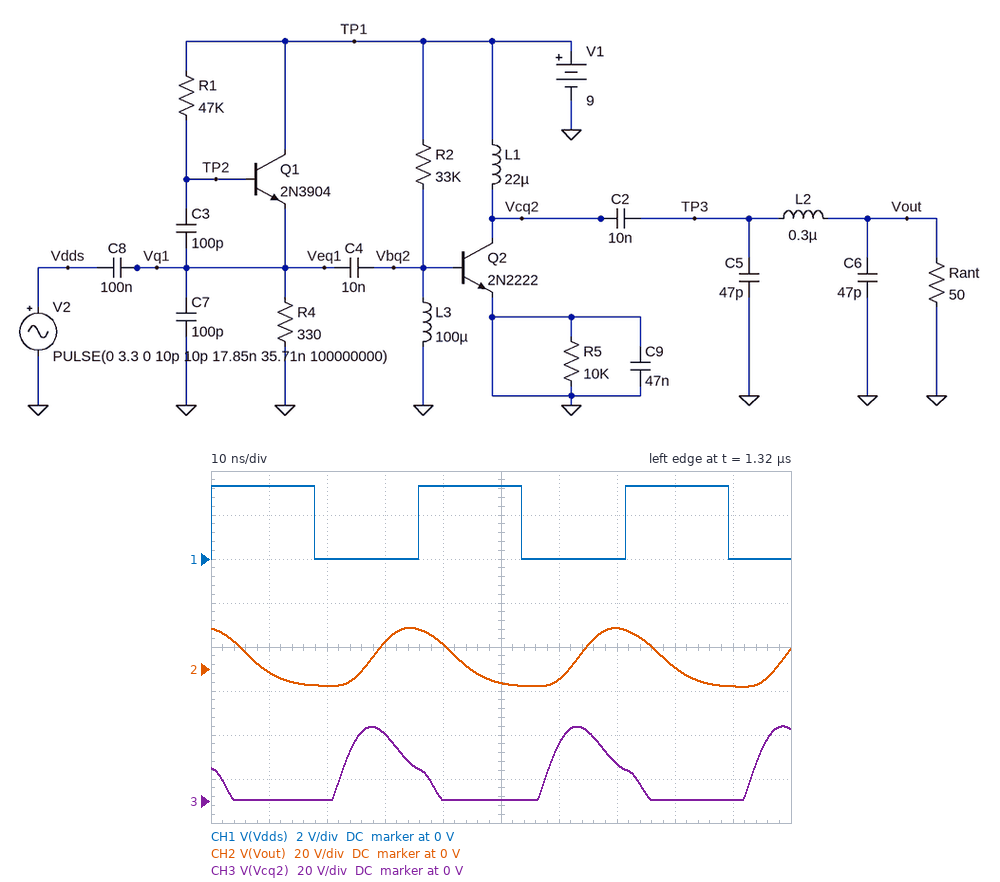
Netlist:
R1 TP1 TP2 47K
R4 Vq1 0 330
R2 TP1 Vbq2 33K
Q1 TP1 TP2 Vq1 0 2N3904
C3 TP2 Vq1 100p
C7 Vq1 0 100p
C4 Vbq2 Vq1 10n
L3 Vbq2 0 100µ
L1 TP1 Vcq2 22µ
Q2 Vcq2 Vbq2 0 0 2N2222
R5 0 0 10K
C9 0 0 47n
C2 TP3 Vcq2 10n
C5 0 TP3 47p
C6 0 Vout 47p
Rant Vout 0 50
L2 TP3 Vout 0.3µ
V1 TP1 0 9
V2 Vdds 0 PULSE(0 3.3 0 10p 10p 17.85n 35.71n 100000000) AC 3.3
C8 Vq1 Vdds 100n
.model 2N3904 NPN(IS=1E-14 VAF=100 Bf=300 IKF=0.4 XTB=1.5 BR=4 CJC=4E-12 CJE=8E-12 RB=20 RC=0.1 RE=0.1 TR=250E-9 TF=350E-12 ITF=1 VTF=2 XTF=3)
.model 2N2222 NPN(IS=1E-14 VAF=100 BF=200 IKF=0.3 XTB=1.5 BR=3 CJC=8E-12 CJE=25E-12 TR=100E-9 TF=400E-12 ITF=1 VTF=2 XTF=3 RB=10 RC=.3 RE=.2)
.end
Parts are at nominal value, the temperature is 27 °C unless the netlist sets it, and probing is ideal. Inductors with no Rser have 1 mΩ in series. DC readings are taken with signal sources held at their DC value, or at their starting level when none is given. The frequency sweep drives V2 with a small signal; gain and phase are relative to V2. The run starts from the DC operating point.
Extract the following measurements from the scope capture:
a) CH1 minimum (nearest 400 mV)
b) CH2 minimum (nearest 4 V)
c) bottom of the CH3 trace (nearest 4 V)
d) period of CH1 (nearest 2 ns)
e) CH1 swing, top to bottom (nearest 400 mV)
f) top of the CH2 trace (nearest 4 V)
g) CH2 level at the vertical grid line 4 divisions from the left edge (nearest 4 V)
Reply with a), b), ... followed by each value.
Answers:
a) 0 V
b) -8 V
c) 0 V
d) 36 ns
e) 3.2 V
f) 20 V
g) 12 V
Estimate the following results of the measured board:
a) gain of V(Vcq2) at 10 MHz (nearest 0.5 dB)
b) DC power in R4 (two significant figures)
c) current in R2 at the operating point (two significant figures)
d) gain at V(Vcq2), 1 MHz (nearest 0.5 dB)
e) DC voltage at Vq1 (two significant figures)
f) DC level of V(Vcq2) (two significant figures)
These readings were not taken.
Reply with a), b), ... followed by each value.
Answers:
a) -39.0 dB
b) 95 mW
c) 270 µA
d) -58.5 dB
e) 5.6 V
f) 9.0 V
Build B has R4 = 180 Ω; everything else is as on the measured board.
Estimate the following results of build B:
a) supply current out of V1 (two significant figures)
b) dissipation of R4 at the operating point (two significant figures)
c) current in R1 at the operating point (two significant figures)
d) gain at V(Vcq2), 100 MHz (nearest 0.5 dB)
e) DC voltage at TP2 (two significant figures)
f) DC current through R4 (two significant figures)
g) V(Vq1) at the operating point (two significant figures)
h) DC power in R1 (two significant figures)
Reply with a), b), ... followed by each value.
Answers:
a) 25 mA
b) 110 mW
c) 82 µA
d) -21.5 dB
e) 5.1 V
f) 24 mA
g) 4.4 V
h) 320 µW
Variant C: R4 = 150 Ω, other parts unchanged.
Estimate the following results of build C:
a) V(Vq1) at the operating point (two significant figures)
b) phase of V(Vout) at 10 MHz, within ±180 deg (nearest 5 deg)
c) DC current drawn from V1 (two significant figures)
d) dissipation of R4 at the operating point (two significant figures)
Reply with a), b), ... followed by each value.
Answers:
a) 4.0 V
b) 75 deg
c) 27 mA
d) 110 mW
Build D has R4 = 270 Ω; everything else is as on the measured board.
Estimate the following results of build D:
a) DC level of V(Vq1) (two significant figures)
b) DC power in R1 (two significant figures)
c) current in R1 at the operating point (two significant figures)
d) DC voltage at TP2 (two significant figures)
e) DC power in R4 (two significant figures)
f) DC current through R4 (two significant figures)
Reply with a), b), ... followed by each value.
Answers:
a) 5.2 V
b) 200 µW
c) 65 µA
d) 5.9 V
e) 100 mW
f) 19 mA
